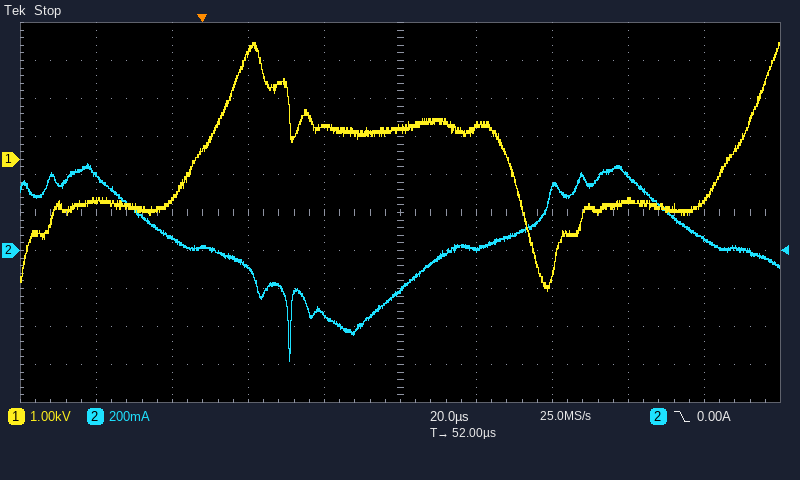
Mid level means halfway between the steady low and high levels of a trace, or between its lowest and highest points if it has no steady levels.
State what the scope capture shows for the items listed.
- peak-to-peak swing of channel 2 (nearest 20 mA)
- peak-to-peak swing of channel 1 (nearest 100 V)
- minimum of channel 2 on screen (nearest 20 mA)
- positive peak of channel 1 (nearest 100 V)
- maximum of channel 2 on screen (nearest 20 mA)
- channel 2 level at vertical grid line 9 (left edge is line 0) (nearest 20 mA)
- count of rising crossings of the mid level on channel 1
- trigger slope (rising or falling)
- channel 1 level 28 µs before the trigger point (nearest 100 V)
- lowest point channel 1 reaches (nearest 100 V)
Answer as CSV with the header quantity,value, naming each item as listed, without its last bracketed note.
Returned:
quantity,value
peak-to-peak swing of channel 2,1.04 A
peak-to-peak swing of channel 1,6.6 kV
minimum of channel 2 on screen,-580 mA
positive peak of channel 1,3.1 kV
maximum of channel 2 on screen,460 mA
channel 2 level at vertical grid line 9 (left edge is line 0),60 mA
count of rising crossings of the mid level on channel 1,2
trigger slope,falling
channel 1 level 28 µs before the trigger point,-1.1 kV
lowest point channel 1 reaches,-3.5 kV
